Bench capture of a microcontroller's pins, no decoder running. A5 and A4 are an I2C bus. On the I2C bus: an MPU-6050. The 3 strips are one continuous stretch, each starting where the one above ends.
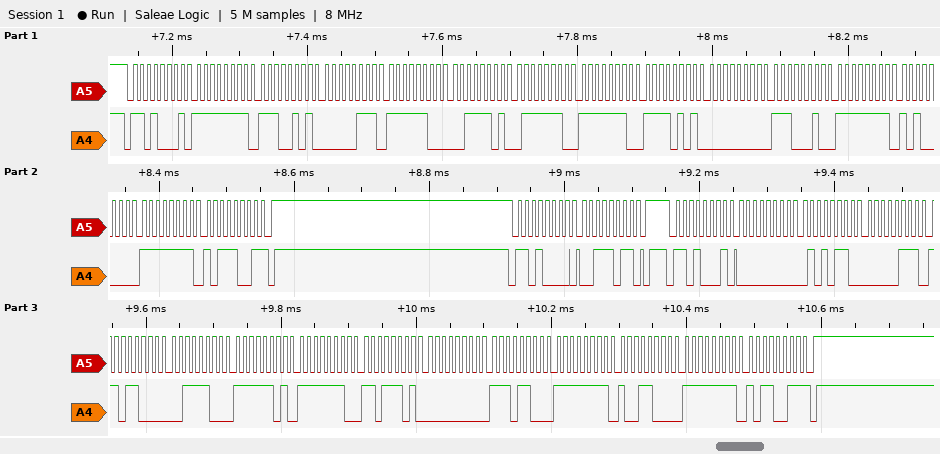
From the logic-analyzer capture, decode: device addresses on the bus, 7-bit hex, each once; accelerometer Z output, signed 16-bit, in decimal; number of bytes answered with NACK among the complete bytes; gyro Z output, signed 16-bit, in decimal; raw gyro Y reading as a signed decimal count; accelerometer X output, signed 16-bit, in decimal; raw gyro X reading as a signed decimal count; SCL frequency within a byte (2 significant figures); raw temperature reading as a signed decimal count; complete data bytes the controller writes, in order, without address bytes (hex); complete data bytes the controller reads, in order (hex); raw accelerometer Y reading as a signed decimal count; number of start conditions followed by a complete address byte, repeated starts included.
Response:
0x68
15613
2
-77
-104
86
236
100 kHz
-291
3B
FF E5 07 FC 3D 7E FE F5 00 E2 FF A0 FF B9 00 56 07 D8 3C FD FE DD 00 EC FF 98 FF B3
2008
3
